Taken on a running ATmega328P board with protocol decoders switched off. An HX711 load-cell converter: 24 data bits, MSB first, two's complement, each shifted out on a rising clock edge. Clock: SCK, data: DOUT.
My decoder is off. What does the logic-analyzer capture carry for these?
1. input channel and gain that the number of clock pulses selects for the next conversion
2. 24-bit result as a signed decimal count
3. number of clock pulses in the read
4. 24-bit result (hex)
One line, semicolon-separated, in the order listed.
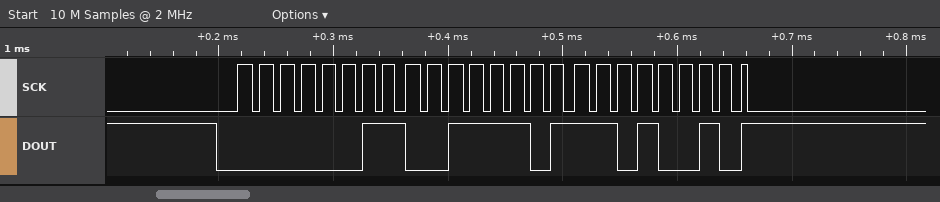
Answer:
channel A, gain 128; 212434; 25; 0x033DD2
